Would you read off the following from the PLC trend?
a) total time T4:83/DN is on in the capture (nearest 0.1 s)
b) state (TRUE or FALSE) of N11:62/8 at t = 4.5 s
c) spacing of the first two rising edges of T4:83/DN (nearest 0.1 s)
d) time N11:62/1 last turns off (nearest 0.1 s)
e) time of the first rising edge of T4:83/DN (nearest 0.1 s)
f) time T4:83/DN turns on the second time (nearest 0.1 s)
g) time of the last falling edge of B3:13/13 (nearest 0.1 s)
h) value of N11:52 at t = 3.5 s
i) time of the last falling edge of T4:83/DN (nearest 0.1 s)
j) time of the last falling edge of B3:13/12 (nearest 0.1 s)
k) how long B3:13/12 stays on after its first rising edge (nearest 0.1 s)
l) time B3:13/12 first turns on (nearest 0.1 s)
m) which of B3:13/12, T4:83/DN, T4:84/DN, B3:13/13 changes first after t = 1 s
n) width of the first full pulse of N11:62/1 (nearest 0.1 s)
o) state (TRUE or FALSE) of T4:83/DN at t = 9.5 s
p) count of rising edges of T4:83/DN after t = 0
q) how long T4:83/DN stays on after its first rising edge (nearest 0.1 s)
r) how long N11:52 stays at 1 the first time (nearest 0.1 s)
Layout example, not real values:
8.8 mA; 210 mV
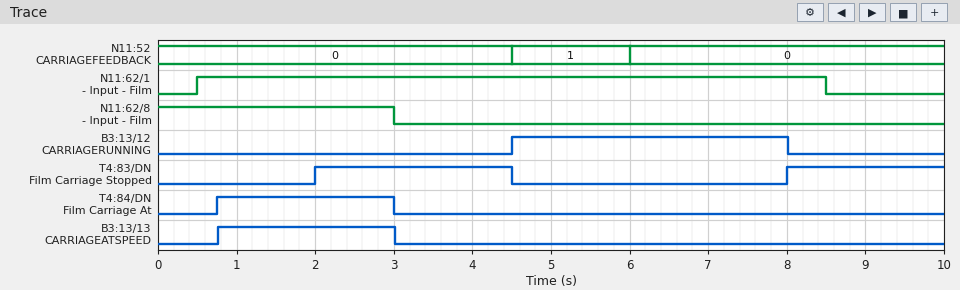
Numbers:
4.5 s; FALSE; 6.0 s; 8.5 s; 2.0 s; 8.0 s; 3.0 s; 0; 4.5 s; 8.0 s; 3.5 s; 4.5 s; T4:83/DN; 8.0 s; TRUE; 2; 2.5 s; 1.5 s
